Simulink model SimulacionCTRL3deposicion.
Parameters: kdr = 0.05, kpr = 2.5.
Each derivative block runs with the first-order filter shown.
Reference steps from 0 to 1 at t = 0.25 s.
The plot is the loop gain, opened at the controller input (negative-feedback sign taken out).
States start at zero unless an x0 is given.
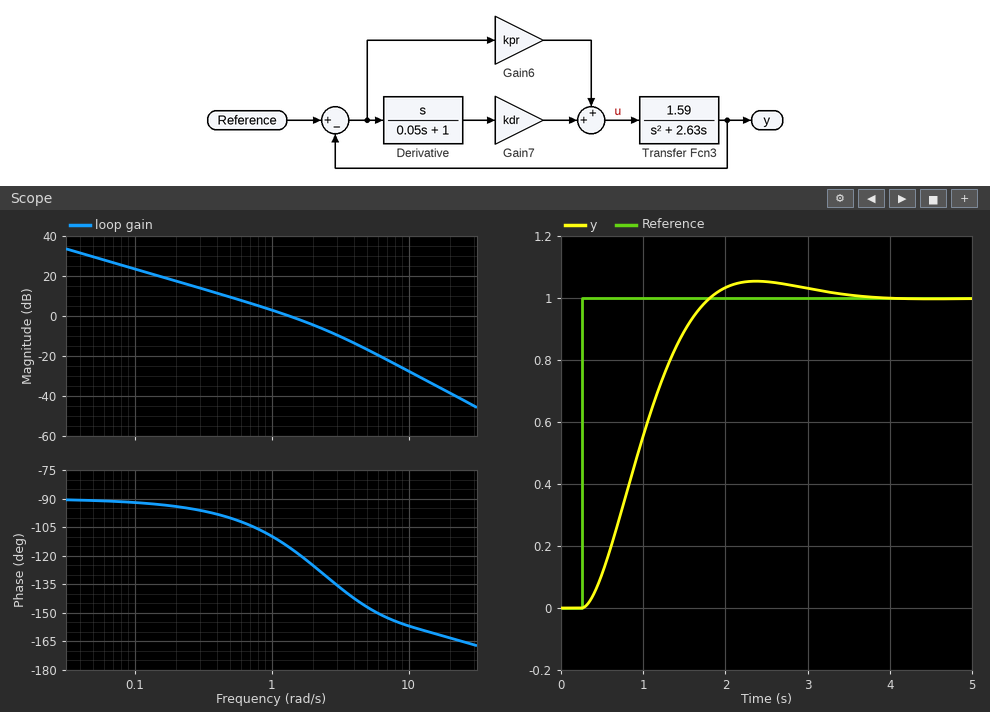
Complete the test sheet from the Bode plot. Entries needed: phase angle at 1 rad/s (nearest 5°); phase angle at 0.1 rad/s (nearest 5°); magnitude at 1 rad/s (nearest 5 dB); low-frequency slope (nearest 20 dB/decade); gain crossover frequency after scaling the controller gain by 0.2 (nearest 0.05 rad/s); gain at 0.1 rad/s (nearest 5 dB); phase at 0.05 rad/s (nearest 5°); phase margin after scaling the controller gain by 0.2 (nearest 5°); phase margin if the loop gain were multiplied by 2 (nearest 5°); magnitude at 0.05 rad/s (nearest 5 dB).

-110°
-90°
5 dB
-20 dB/decade
0.30 rad/s
25 dB
-90°
85°
50°
30 dB
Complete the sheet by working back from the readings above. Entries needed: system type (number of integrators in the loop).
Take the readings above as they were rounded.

1
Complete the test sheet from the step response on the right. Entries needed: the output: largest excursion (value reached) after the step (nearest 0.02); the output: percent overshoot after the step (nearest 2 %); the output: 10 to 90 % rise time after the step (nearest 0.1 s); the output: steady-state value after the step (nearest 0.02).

1.06
6 %
1.0 s
1.00
